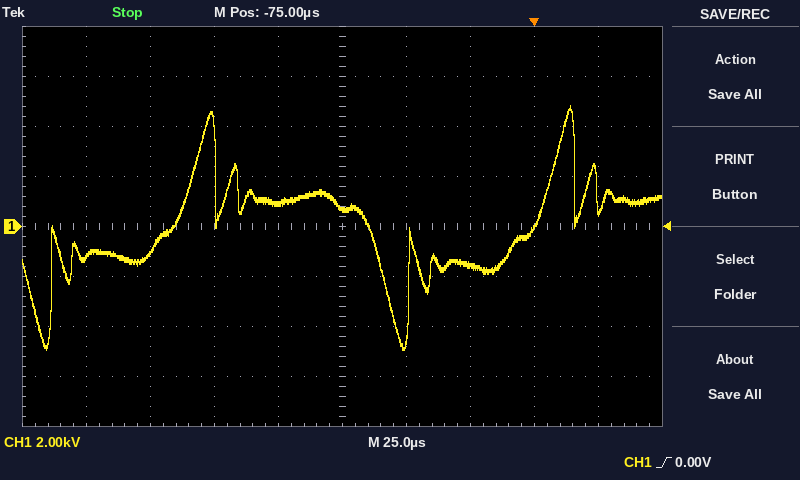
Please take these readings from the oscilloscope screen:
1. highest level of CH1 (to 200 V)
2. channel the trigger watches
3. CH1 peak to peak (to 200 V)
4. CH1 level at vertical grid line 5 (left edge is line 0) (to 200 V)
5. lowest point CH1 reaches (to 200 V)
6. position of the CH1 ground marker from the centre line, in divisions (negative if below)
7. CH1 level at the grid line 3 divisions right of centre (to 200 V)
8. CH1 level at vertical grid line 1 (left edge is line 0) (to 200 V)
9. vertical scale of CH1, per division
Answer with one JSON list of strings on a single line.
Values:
["4.8 kV", "CH1", "9.8 kV", "800 V", "-5.0 kV", "0.0 div", "0.0 kV", "-1.2 kV", "2 kV"]
